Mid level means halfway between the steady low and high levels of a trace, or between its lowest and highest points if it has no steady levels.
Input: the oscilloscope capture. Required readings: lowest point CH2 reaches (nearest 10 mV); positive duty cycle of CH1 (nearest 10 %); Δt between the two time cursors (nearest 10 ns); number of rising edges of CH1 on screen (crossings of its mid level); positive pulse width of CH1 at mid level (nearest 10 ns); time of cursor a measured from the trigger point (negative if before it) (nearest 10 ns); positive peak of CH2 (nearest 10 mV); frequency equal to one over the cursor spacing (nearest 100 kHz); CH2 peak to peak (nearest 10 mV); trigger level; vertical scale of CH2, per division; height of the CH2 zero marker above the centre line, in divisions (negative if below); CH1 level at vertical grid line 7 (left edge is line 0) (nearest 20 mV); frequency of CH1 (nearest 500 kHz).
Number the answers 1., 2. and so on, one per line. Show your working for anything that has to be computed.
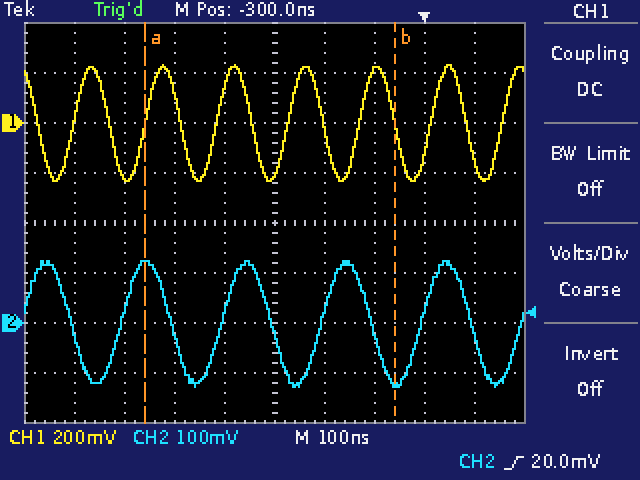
1. -130 mV
2. 50 %
3. 500 ns
4. 7
5. 70 ns
6. -560 ns
7. 120 mV
8. 1 / 500 ns ≈ 2.0 MHz
9. 120 mV − (-130 mV) = 250 mV
10. 20.0 mV
11. 100 mV
12. -2.0 div
13. 200 mV
14. 7.0 MHz
